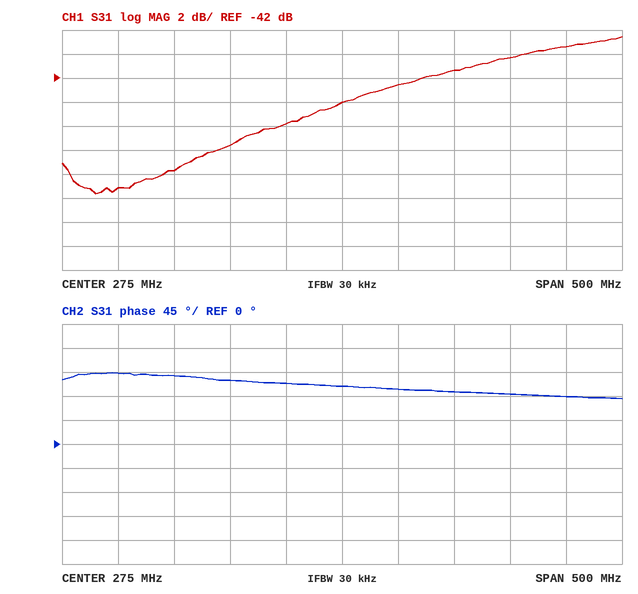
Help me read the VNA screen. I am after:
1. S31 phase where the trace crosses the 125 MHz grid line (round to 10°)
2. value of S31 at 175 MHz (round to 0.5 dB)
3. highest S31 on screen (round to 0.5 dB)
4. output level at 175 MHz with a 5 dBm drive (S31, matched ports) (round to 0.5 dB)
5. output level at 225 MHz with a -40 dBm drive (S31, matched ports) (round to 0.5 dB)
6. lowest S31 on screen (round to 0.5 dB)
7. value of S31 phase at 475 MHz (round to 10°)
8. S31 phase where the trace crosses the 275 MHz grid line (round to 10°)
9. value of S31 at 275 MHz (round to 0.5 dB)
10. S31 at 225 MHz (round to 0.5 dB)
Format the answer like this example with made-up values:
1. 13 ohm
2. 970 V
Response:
1. 130°
2. -47.5 dB
3. -38.5 dB
4. -42.5 dBm
5. -86.0 dBm
6. -51.5 dB
7. 90°
8. 110°
9. -44.0 dB
10. -46.0 dB
